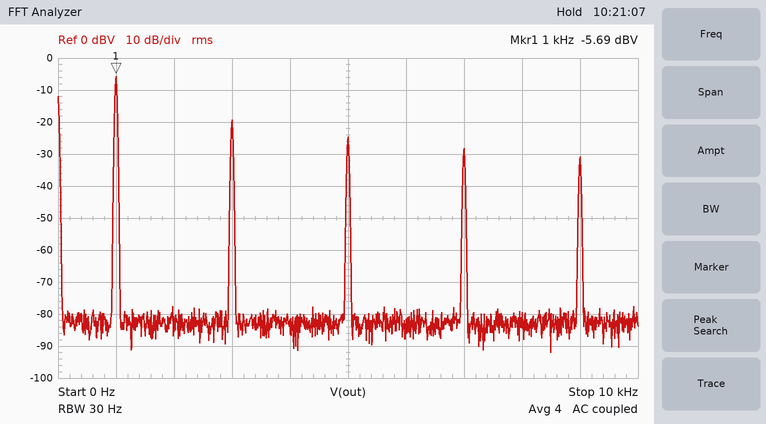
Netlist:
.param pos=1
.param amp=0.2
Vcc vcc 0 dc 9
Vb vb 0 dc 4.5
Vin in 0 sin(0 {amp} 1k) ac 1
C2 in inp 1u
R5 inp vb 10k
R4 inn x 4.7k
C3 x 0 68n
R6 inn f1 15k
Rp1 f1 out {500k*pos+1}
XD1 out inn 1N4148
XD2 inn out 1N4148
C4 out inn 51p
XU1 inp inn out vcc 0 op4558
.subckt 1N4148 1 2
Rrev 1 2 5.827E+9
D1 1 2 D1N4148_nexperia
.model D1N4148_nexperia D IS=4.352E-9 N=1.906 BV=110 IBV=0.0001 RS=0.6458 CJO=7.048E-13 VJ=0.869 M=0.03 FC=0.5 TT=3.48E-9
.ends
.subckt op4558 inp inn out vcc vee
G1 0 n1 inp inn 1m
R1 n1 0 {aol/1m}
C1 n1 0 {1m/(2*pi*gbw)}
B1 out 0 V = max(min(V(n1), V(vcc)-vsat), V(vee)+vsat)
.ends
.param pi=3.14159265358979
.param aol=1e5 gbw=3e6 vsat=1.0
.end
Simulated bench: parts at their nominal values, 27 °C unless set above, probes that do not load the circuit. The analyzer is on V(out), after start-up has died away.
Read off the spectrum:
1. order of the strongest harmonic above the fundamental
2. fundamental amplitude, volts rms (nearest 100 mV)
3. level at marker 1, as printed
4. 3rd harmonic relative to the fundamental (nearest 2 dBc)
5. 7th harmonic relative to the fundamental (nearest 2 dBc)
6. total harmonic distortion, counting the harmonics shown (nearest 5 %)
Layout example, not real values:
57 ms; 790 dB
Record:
3; 500 mV; -5.69 dBV; -14 dBc; -22 dBc; 25 %
